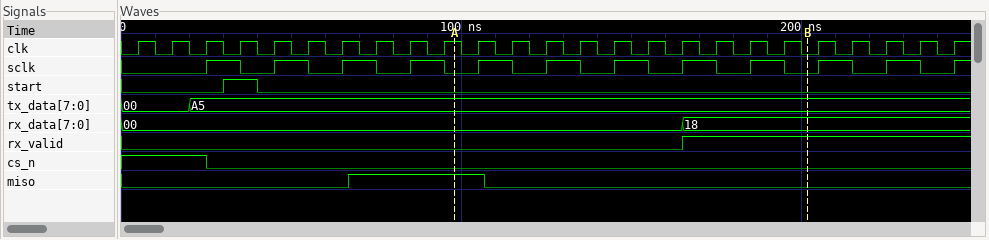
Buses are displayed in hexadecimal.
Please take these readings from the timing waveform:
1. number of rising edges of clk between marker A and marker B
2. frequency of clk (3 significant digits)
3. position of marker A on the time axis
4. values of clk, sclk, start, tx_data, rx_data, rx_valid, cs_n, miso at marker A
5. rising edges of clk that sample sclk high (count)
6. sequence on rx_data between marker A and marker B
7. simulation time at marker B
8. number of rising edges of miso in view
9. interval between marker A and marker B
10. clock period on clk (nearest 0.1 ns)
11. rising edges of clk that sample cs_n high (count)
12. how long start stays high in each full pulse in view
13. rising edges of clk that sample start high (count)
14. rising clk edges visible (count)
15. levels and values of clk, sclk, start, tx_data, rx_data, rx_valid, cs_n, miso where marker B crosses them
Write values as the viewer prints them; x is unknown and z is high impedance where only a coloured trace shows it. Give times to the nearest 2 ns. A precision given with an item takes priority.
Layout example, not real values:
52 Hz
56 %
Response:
10
100 MHz
98 ns
clk=1, sclk=0, start=0, tx_data=A5, rx_data=00, rx_valid=0, cs_n=0, miso=1
11
00, 18
202 ns
1
104 ns
10 ns
3
10 ns
1
25
clk=0, sclk=0, start=0, tx_data=A5, rx_data=18, rx_valid=1, cs_n=0, miso=0
